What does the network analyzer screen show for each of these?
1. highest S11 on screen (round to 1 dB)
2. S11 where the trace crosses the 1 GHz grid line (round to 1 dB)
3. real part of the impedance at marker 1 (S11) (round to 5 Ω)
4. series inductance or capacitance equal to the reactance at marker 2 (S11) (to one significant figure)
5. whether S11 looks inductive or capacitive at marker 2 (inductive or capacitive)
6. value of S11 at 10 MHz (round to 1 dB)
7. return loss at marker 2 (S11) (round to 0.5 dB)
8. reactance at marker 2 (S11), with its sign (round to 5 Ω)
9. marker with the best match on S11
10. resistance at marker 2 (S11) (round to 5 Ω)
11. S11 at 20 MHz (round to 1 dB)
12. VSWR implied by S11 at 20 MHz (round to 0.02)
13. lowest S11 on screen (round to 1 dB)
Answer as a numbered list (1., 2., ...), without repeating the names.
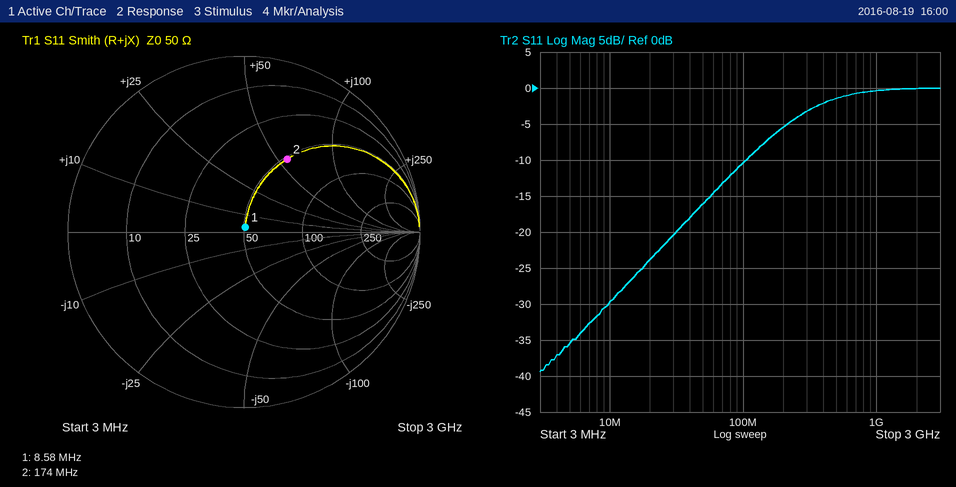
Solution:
1. 0 dB
2. 0 dB
3. 50 Ω
4. 50 nH
5. inductive
6. -30 dB
7. 6.5 dB
8. +55 Ω
9. marker 1
10. 50 Ω
11. -24 dB
12. 1.14
13. -39 dB
